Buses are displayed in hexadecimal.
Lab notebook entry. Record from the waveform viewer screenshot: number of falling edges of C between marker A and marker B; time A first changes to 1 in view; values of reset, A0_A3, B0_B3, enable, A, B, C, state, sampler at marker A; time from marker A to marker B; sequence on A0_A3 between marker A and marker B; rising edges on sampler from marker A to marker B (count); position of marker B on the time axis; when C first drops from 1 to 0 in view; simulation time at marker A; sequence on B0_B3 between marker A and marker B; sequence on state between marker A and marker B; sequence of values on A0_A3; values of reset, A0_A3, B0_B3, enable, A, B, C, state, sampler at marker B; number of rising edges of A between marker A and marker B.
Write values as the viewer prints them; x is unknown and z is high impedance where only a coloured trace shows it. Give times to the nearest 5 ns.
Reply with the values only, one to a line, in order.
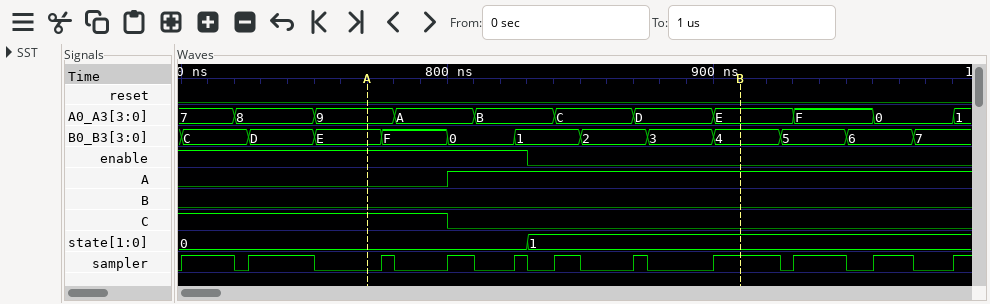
1
800 ns
reset=0, A0_A3=9, B0_B3=E, enable=1, A=0, B=0, C=1, state=0, sampler=0
140 ns
9, A, B, C, D, E
6
910 ns
800 ns
770 ns
E, F, 0, 1, 2, 3, 4
0, 1
7, 8, 9, A, B, C, D, E, F, 0, 1
reset=0, A0_A3=E, B0_B3=4, enable=0, A=1, B=0, C=0, state=1, sampler=1
1
